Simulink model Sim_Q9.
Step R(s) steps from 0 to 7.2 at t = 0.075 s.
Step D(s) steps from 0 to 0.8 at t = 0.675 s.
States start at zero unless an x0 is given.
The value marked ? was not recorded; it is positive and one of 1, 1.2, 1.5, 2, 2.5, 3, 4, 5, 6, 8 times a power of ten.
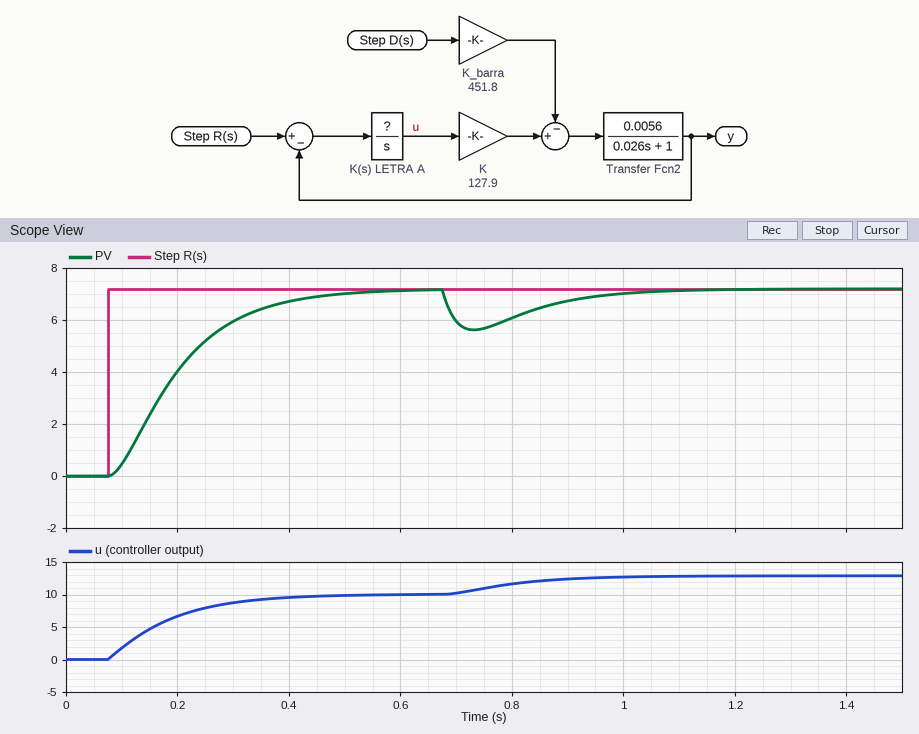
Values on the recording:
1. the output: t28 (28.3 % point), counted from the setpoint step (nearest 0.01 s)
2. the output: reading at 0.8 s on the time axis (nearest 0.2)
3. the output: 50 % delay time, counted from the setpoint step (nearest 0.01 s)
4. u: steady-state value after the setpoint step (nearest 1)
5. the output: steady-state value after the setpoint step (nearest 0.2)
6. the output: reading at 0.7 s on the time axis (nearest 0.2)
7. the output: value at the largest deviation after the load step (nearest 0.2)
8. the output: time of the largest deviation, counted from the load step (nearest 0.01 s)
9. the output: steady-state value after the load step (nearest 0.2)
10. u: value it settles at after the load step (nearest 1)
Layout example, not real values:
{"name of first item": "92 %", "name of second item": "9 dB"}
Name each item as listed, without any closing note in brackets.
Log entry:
{"the output: t28 (28.3 % point), counted from the setpoint step": "0.07 s", "the output: reading at 0.8 s on the time axis": "6.0", "the output: 50 % delay time, counted from the setpoint step": "0.11 s", "u: steady-state value after the setpoint step": "10", "the output: steady-state value after the setpoint step": "7.2", "the output: reading at 0.7 s on the time axis": "6.0", "the output: value at the largest deviation after the load step": "5.6", "the output: time of the largest deviation, counted from the load step": "0.06 s", "the output: steady-state value after the load step": "7.2", "u: value it settles at after the load step": "13"}
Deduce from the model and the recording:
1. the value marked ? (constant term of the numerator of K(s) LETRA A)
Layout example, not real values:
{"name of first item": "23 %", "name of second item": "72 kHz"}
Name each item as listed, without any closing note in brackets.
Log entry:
{"the value marked ? (constant term of the numerator of K(s) LETRA A)": "10"}
